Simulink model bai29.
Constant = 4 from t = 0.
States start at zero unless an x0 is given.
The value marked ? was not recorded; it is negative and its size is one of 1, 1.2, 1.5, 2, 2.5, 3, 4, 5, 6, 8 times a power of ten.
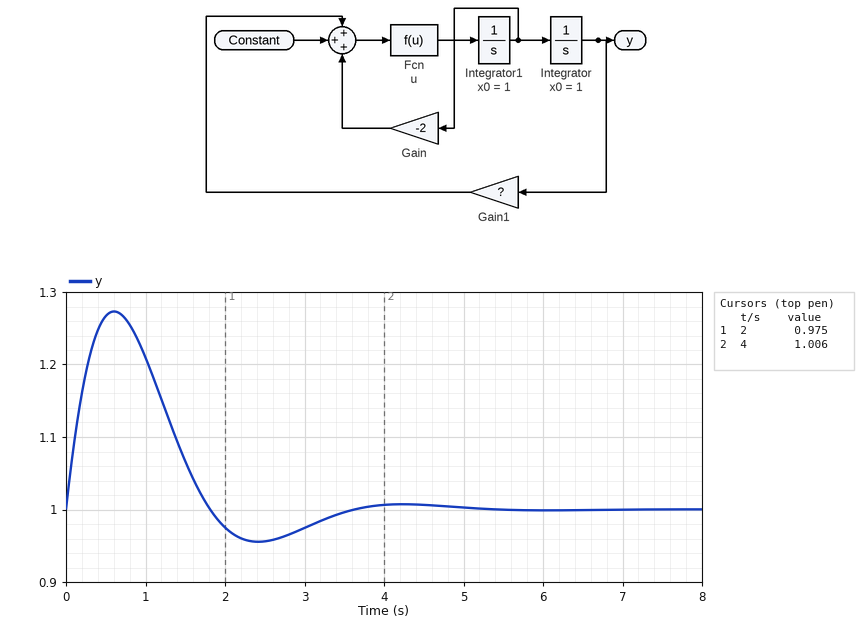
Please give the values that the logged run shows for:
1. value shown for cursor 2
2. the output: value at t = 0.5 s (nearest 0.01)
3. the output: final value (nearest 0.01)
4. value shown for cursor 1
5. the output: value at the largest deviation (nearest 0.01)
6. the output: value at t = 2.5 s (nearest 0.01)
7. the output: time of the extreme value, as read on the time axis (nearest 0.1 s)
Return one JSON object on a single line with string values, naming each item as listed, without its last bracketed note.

{"value shown for cursor 2": "1.006", "the output: value at t = 0.5 s": "1.27", "the output: final value": "1.00", "value shown for cursor 1": "0.975", "the output: value at the largest deviation": "1.27", "the output: value at t = 2.5 s": "0.96", "the output: time of the extreme value, as read on the time axis": "0.6 s"}
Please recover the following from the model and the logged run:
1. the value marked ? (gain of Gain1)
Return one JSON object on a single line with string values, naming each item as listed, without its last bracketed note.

{"the value marked ?": "-4"}
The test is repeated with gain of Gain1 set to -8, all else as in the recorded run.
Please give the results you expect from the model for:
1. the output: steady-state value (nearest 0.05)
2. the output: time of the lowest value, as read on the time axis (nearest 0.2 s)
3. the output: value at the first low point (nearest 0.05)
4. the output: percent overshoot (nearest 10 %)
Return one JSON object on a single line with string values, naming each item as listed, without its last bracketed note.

{"the output: steady-state value": "0.50", "the output: time of the lowest value, as read on the time axis": "1.4 s", "the output: value at the first low point": "0.30", "the output: percent overshoot": "40 %"}
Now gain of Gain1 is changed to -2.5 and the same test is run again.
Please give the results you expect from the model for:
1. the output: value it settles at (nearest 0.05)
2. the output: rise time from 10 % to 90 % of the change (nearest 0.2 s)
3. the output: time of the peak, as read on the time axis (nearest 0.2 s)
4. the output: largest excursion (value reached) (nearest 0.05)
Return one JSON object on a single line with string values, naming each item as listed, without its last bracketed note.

{"the output: value it settles at": "1.60", "the output: rise time from 10 % to 90 % of the change": "0.6 s", "the output: time of the peak, as read on the time axis": "1.6 s", "the output: largest excursion (value reached)": "1.70"}
